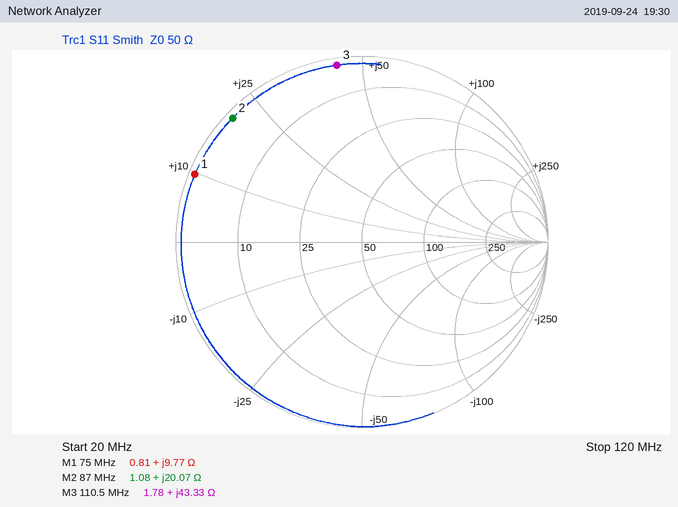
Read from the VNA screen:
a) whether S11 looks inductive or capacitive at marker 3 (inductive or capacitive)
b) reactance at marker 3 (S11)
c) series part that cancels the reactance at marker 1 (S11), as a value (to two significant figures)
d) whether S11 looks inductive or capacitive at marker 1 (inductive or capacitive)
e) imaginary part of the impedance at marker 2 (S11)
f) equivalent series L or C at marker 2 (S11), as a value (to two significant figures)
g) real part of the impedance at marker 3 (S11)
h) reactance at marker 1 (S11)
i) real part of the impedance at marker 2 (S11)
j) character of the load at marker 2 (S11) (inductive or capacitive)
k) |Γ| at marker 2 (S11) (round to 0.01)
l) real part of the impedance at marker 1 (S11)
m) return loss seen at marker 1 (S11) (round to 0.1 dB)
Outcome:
inductive
+43.33 Ω
220 pF
inductive
+20.07 Ω
37 nH
1.78 Ω
+9.77 Ω
1.08 Ω
inductive
0.96
0.81 Ω
0.3 dB
